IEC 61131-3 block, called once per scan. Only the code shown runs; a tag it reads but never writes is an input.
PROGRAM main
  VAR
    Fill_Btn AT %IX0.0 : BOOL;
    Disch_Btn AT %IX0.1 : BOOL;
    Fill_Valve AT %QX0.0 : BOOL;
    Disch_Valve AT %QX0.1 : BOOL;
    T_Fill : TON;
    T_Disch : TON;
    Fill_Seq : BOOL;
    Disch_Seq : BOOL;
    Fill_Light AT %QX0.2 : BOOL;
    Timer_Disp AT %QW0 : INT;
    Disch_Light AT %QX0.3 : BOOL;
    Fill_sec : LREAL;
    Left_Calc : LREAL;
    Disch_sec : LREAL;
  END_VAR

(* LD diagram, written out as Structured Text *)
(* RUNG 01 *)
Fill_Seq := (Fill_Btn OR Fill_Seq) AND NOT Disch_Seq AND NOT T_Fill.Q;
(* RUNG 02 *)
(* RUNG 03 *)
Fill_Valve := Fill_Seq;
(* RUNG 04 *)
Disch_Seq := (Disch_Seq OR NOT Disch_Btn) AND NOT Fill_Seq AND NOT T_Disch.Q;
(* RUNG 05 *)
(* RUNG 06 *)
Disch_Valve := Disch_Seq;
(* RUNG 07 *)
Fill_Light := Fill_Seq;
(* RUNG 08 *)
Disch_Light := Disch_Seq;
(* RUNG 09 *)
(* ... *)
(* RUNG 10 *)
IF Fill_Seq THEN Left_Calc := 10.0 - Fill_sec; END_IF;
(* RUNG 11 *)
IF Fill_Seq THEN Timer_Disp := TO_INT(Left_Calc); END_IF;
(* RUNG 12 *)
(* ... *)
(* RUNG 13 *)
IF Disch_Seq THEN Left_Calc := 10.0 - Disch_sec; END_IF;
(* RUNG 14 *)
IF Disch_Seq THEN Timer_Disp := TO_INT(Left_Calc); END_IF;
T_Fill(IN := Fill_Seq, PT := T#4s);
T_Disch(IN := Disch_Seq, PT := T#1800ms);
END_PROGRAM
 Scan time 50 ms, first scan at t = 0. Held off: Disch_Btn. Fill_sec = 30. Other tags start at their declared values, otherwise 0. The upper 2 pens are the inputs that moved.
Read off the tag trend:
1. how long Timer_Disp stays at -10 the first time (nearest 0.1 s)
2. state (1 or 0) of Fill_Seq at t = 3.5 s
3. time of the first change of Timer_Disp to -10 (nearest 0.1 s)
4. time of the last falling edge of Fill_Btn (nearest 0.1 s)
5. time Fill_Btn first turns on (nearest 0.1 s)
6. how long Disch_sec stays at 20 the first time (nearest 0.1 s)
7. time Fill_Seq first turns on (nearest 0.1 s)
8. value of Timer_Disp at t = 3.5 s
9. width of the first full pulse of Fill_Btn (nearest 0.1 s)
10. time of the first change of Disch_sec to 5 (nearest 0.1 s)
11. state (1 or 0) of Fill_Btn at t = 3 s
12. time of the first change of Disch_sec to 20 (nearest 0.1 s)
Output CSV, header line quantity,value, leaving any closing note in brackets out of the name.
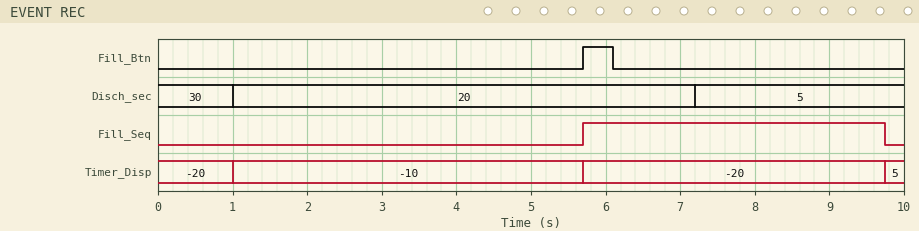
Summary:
quantity,value
how long Timer_Disp stays at -10 the first time,4.7 s
state (1 or 0) of Fill_Seq at t = 3.5 s,0
time of the first change of Timer_Disp to -10,1.0 s
time of the last falling edge of Fill_Btn,6.1 s
time Fill_Btn first turns on,5.7 s
how long Disch_sec stays at 20 the first time,6.2 s
time Fill_Seq first turns on,5.7 s
value of Timer_Disp at t = 3.5 s,-10
width of the first full pulse of Fill_Btn,0.4 s
time of the first change of Disch_sec to 5,7.2 s
state (1 or 0) of Fill_Btn at t = 3 s,0
time of the first change of Disch_sec to 20,1.0 s
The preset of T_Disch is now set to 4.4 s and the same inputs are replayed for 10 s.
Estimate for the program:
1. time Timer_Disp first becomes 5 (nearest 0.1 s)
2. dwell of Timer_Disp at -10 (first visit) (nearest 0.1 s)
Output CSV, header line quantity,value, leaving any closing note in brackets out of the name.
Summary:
quantity,value
time Timer_Disp first becomes 5,7.2 s
dwell of Timer_Disp at -10 (first visit),6.2 s
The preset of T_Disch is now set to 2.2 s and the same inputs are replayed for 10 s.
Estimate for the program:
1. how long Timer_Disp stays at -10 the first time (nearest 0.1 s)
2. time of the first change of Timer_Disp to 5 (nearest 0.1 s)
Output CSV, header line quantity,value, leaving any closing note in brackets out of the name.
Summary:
quantity,value
how long Timer_Disp stays at -10 the first time,6.2 s
time of the first change of Timer_Disp to 5,7.2 s
